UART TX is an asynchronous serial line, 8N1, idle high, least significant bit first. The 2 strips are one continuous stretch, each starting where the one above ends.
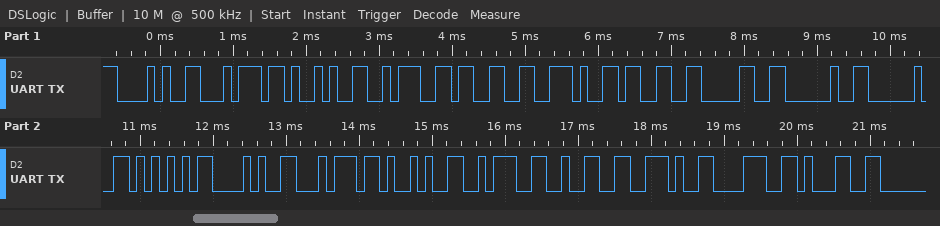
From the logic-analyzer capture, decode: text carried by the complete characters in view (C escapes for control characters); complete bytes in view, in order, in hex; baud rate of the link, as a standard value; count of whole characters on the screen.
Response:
"(t):3.30  U(t):2.81"
28 74 29 3A 33 2E 33 30 20 20 55 28 74 29 3A 32 2E 38 31
9600 baud
19
